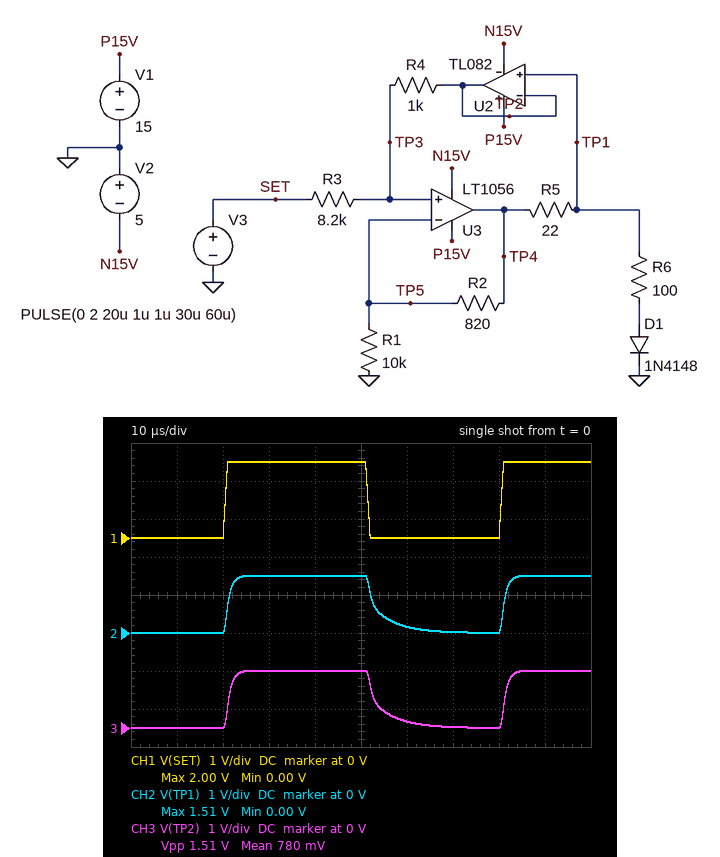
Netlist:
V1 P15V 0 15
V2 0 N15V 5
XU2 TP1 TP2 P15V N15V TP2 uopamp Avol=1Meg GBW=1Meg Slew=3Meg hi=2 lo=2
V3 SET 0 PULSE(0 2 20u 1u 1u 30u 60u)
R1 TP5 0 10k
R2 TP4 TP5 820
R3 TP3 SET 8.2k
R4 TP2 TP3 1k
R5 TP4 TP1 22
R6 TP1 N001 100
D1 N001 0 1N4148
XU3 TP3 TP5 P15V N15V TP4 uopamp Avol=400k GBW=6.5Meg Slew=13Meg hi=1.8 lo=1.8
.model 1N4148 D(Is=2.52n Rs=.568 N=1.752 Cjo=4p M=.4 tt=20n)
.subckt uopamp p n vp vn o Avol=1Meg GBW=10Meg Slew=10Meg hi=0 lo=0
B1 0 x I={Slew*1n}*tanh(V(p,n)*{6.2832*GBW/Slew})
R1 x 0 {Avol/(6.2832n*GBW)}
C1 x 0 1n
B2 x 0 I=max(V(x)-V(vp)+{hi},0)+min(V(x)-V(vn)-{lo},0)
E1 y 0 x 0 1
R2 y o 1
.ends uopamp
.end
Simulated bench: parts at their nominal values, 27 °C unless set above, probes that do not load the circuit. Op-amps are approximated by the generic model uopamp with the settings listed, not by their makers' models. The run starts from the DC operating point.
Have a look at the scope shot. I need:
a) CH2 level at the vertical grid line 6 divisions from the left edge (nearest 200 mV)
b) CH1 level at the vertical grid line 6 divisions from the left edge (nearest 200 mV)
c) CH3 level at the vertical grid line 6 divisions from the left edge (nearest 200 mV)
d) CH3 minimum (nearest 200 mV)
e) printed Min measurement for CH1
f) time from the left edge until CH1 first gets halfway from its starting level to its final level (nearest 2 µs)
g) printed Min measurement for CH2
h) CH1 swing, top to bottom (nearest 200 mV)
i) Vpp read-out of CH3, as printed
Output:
200 mV
0 V
200 mV
0 V
0.00 V
20 µs
0.00 V
2.0 V
1.51 V
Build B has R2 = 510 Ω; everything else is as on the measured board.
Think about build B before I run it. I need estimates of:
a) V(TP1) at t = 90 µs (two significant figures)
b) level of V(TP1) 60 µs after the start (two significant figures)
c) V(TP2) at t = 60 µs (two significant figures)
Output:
1.3 V
49 mV
52 mV
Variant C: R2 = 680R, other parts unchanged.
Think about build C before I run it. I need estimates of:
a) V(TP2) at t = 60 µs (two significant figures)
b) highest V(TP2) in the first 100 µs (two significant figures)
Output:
100 mV
1.4 V
